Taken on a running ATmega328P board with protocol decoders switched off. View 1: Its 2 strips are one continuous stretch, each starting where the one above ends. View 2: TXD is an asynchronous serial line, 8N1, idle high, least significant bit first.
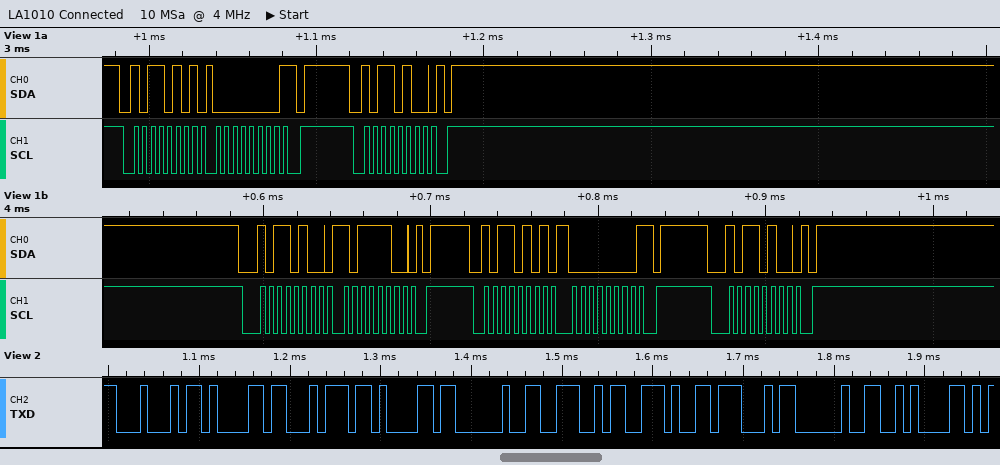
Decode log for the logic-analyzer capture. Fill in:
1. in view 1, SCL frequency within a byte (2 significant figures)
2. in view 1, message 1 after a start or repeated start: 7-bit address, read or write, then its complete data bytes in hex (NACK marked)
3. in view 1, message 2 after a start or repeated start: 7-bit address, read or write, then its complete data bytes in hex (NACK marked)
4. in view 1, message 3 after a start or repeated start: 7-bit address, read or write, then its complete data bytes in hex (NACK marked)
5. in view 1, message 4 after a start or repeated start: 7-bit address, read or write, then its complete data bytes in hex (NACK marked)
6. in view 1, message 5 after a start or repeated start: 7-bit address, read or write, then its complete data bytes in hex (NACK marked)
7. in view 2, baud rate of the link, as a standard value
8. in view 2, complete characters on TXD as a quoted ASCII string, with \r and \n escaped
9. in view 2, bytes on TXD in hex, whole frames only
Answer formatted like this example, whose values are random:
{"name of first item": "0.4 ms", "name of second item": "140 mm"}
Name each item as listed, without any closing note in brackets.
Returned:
{"in view 1, SCL frequency within a byte": "200 kHz", "in view 1, message 1 after a start or repeated start: 7-bit address, read or write, then its complete data bytes in hex": "0x5A read: 00 NACK", "in view 1, message 2 after a start or repeated start: 7-bit address, read or write, then its complete data bytes in hex": "0x5A write", "in view 1, message 3 after a start or repeated start: 7-bit address, read or write, then its complete data bytes in hex": "0x5A write: BC", "in view 1, message 4 after a start or repeated start: 7-bit address, read or write, then its complete data bytes in hex": "0x5A read: 00 NACK", "in view 1, message 5 after a start or repeated start: 7-bit address, read or write, then its complete data bytes in hex": "0x5A write", "in view 2, baud rate of the link, as a standard value": "115200 baud", "in view 2, complete characters on TXD as a quoted ASCII string, with \\r and \\n escaped": "\"Data N.G \\n\"", "in view 2, bytes on TXD in hex, whole frames only": "44 61 74 61 20 4E 2E 47 20 0A"}
